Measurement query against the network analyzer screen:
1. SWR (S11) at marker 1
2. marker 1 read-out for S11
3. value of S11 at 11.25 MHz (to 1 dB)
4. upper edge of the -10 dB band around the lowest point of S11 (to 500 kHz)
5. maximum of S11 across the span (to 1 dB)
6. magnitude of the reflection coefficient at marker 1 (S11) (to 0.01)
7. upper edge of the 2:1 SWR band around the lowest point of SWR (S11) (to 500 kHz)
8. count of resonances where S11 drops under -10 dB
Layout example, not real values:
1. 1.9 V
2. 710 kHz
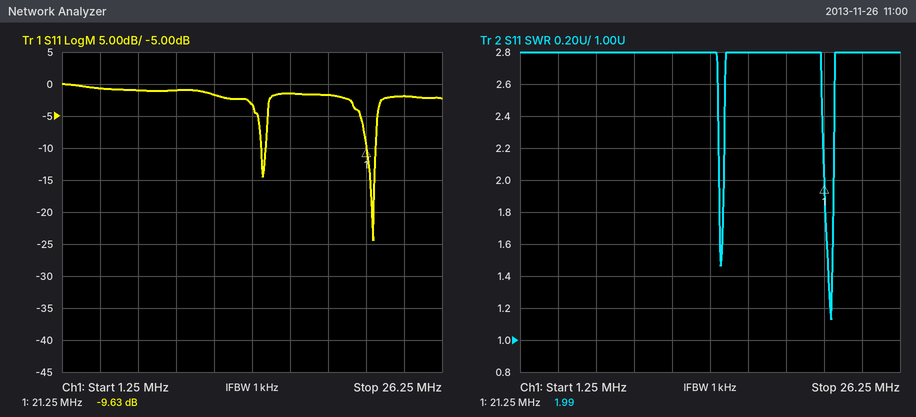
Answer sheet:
1. 1.99
2. -9.63 dB
3. -2 dB
4. 22.0 MHz
5. 0 dB
6. 0.33
7. 22.0 MHz
8. 2
